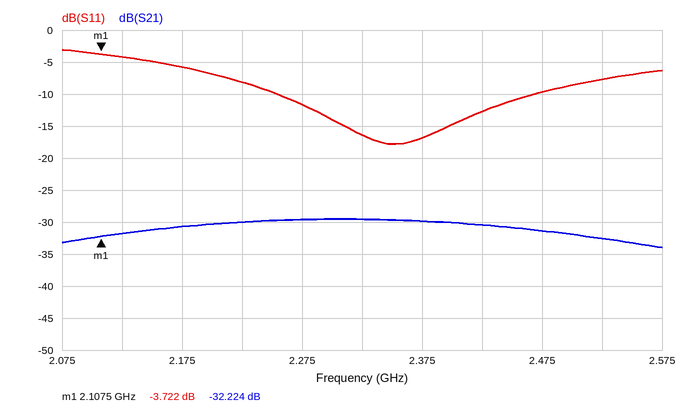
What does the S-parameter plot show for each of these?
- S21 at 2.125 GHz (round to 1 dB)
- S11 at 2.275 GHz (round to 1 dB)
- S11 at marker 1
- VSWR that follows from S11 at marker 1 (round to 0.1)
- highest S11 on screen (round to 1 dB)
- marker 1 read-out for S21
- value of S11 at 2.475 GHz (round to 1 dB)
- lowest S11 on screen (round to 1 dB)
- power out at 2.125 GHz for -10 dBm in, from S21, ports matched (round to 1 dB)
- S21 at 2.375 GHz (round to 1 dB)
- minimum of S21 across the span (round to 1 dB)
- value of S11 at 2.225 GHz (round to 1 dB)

-32 dB
-12 dB
-3.722 dB
4.7
-3 dB
-32.224 dB
-10 dB
-18 dB
-42 dBm
-30 dB
-34 dB
-8 dB
